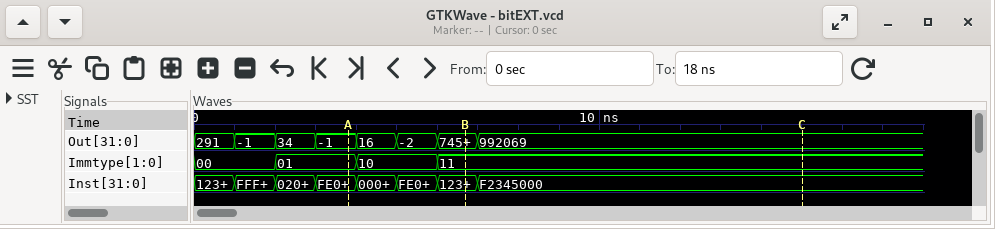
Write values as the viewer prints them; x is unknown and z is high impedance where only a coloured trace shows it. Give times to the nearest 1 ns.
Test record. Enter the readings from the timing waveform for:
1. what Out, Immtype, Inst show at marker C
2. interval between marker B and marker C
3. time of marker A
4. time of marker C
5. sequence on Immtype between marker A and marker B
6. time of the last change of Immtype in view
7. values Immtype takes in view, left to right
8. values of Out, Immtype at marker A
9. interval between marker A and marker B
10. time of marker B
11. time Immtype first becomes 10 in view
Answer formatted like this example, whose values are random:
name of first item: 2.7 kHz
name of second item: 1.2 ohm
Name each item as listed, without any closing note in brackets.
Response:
what Out, Immtype, Inst show at marker C: Out=992069, Immtype=11, Inst=F2345000
interval between marker B and marker C: 8 ns
time of marker A: 4 ns
time of marker C: 15 ns
sequence on Immtype between marker A and marker B: 01, 10, 11
time of the last change of Immtype in view: 6 ns
values Immtype takes in view, left to right: 00, 01, 10, 11
values of Out, Immtype at marker A: Out=-1, Immtype=01
interval between marker A and marker B: 3 ns
time of marker B: 7 ns
time Immtype first becomes 10 in view: 4 ns
